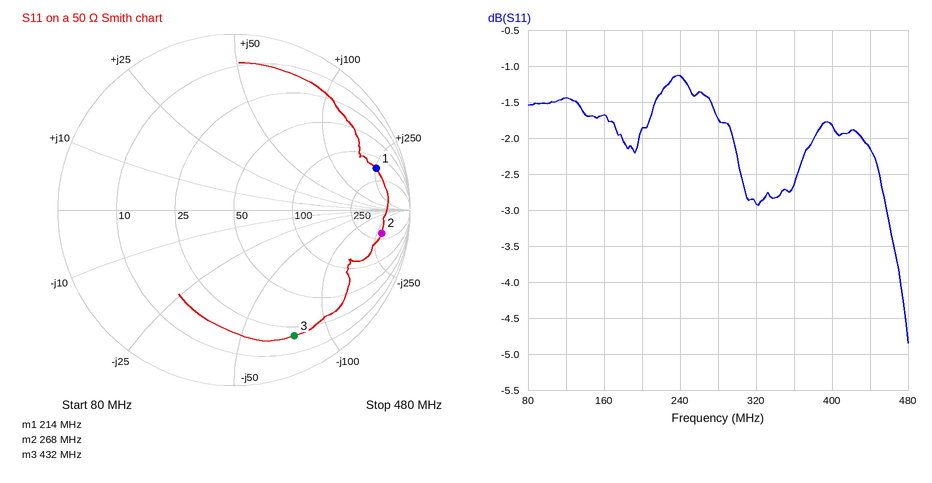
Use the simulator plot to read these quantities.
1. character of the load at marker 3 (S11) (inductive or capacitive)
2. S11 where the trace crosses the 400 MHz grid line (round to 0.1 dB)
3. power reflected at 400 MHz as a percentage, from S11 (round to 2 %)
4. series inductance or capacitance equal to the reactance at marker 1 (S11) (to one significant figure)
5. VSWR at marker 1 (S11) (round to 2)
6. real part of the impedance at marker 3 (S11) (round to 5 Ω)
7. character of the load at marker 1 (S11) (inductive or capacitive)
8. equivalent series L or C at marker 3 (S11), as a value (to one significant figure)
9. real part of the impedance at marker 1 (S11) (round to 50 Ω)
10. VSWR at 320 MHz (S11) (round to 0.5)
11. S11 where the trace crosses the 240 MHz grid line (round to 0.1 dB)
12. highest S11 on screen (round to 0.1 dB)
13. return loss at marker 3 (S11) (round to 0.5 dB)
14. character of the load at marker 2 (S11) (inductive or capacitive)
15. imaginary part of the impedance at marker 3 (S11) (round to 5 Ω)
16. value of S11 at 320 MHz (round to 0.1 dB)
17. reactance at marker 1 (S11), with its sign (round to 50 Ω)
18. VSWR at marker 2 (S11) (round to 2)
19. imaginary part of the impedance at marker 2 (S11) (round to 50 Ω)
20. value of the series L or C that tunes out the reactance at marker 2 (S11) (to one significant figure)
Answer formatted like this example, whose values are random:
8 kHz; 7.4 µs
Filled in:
capacitive; -1.8 dB; 66 %; 200 nH; 12; 20 Ω; inductive; 5 pF; 150 Ω; 6.0; -1.1 dB; -1.1 dB; 2.0 dB; capacitive; -75 Ω; -2.9 dB; +250 Ω; 12; -300 Ω; 200 nH
